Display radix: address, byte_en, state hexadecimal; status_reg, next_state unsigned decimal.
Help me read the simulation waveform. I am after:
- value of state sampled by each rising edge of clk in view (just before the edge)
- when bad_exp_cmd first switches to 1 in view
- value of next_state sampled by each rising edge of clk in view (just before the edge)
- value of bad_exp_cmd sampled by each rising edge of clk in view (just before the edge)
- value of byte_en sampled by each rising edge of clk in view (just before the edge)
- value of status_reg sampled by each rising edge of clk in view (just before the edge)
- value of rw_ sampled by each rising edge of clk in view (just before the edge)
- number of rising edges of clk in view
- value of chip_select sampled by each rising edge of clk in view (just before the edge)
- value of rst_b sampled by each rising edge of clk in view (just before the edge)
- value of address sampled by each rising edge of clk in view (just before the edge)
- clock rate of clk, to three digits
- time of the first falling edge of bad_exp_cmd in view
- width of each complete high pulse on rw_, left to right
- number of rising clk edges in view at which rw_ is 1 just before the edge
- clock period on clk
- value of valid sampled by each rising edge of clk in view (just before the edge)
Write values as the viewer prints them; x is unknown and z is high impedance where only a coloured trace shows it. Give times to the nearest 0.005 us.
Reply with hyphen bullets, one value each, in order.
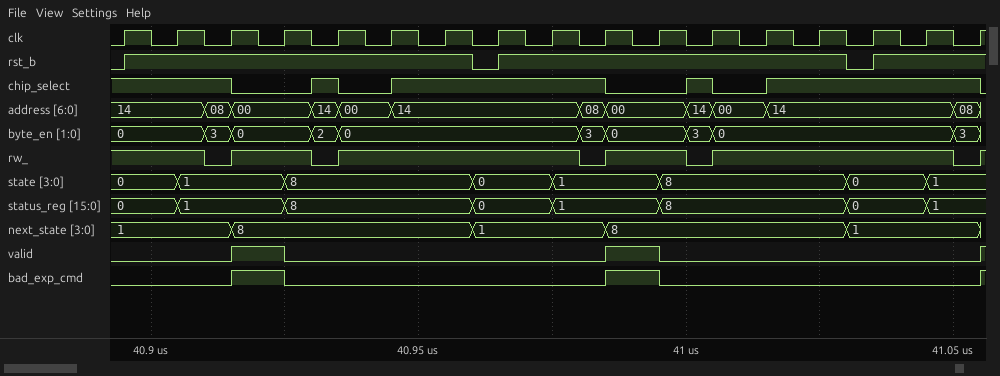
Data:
- 0, 0, 1, 1, 8, 8, 8, 0, 0, 1, 1, 8, 8, 8, 0, 0, 1
- 40.915 us
- 1, 1, 1, 8, 8, 8, 8, 1, 1, 1, 8, 8, 8, 8, 1, 1, 1
- 0 0 0 1 0 0 0 0 0 0 1 0 0 0 0 0 0
- 0, 0, 3, 0, 2, 0, 0, 0, 0, 3, 0, 3, 0, 0, 0, 0, 3
- 0, 0, 1, 1, 8, 8, 8, 0, 0, 1, 1, 8, 8, 8, 0, 0, 1
- 1 1 0 1 0 1 1 1 1 0 1 0 1 1 1 1 0
- 17
- 1 1 1 0 1 0 1 1 1 1 0 1 0 1 1 1 1
- 0 1 1 1 1 1 1 0 1 1 1 1 1 1 0 1 1
- 14, 14, 08, 00, 14, 00, 14, 14, 14, 08, 00, 14, 00, 14, 14, 14, 08
- 100 MHz
- 40.925 us
- 0.015 us, 0.045 us, 0.015 us, 0.045 us
- 12
- 0.01 us
- 0 0 0 1 0 0 0 0 0 0 1 0 0 0 0 0 0
